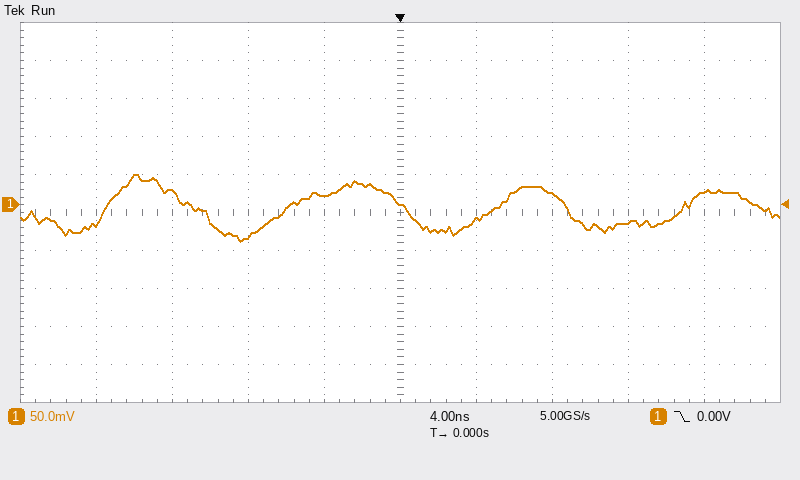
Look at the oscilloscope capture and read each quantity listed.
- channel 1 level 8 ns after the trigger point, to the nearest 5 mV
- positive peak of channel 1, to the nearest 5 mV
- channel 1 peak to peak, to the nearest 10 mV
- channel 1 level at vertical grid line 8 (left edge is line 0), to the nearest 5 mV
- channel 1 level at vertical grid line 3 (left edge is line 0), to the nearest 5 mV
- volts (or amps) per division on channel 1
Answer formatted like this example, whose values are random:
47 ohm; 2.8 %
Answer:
15 mV; 40 mV; 90 mV; -20 mV; -40 mV; 50 mV
